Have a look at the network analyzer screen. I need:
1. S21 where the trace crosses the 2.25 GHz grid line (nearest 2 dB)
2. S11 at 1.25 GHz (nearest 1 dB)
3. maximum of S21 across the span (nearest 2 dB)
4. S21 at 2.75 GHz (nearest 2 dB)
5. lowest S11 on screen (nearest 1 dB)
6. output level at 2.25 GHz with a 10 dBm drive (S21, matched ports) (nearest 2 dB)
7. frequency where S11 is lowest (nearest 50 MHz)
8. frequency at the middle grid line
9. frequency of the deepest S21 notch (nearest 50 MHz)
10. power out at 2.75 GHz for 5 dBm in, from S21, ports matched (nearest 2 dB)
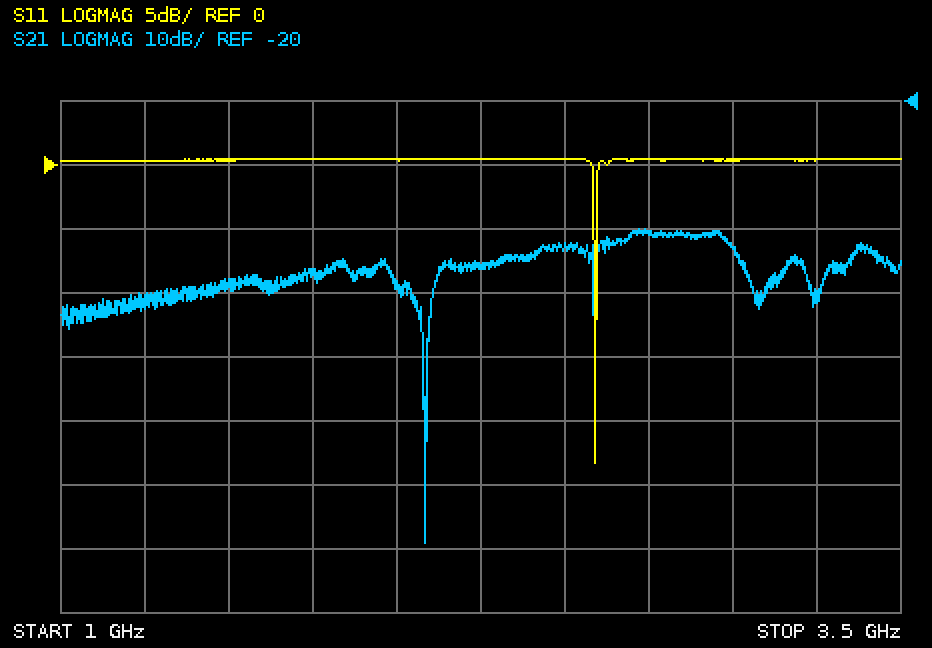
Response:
-46 dB
0 dB
-40 dB
-40 dB
-23 dB
-36 dBm
2.60 GHz
2.25 GHz
2.10 GHz
-36 dBm
